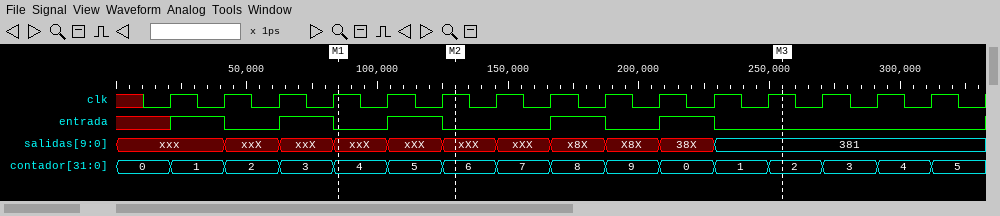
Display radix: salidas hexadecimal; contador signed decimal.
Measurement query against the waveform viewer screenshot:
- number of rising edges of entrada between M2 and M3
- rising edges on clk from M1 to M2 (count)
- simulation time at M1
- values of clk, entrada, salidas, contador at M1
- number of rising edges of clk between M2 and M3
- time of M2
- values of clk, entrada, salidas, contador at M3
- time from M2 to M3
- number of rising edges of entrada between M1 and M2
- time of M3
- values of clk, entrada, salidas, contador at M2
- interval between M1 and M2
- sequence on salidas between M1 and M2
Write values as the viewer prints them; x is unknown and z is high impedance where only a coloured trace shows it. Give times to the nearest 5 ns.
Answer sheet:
2
2
85 ns
clk=1, entrada=0, salidas=xxX, contador=4
6
130 ns
clk=1, entrada=0, salidas=381, contador=2
125 ns
1
255 ns
clk=1, entrada=0, salidas=xXX, contador=6
45 ns
xxX, xXX, xXX
